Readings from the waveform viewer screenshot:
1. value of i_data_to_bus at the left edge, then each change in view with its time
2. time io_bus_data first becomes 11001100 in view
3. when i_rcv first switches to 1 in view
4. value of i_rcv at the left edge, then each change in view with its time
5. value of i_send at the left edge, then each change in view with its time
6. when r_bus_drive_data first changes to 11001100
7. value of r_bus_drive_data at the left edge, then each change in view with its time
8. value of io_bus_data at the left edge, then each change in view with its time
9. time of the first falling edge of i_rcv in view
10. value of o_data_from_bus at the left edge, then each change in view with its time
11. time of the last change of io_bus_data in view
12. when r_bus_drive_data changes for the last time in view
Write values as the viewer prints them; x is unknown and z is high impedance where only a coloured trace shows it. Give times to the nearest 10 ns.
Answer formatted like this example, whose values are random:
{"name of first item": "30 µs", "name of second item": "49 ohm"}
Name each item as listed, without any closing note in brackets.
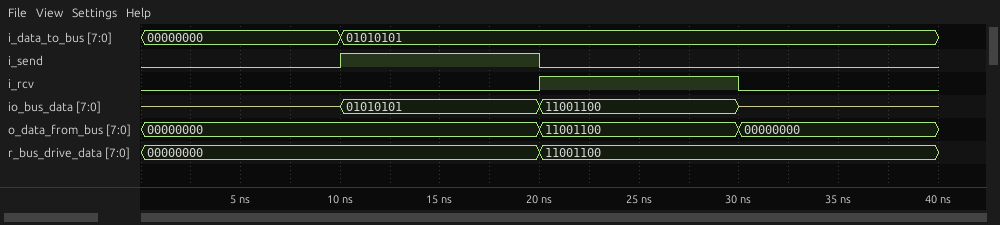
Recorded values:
{"value of i_data_to_bus at the left edge, then each change in view with its time": "00000000, 01010101 at 10 ns", "time io_bus_data first becomes 11001100 in view": "20 ns", "when i_rcv first switches to 1 in view": "20 ns", "value of i_rcv at the left edge, then each change in view with its time": "0, 1 at 20 ns, 0 at 30 ns", "value of i_send at the left edge, then each change in view with its time": "0, 1 at 10 ns, 0 at 20 ns", "when r_bus_drive_data first changes to 11001100": "20 ns", "value of r_bus_drive_data at the left edge, then each change in view with its time": "00000000, 11001100 at 20 ns", "value of io_bus_data at the left edge, then each change in view with its time": "z, 01010101 at 10 ns, 11001100 at 20 ns, z at 30 ns", "time of the first falling edge of i_rcv in view": "30 ns", "value of o_data_from_bus at the left edge, then each change in view with its time": "00000000, 11001100 at 20 ns, 00000000 at 30 ns", "time of the last change of io_bus_data in view": "30 ns", "when r_bus_drive_data changes for the last time in view": "20 ns"}
